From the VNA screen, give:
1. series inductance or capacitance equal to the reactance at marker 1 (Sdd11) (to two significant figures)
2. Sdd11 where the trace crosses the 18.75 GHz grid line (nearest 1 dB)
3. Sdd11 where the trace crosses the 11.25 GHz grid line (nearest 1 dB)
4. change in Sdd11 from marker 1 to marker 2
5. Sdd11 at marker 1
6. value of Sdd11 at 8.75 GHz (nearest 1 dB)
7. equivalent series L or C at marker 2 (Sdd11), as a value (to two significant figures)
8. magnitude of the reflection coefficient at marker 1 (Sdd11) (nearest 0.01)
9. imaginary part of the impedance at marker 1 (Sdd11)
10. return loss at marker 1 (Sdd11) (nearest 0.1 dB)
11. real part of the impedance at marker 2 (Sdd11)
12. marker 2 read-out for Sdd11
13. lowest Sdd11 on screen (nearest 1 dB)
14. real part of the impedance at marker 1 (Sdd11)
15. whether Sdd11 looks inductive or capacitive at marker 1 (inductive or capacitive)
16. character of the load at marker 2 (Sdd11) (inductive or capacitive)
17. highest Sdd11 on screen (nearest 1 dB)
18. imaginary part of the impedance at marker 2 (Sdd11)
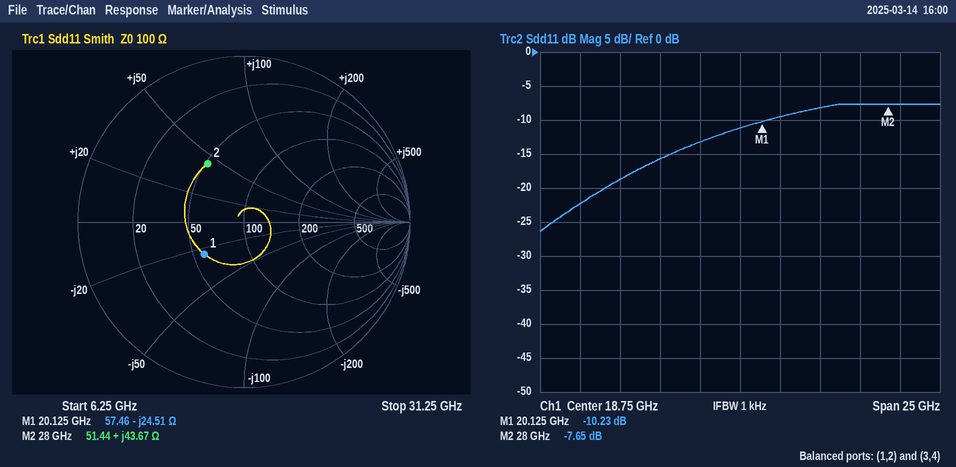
320 fF
-11 dB
-19 dB
2.58 dB
-10.23 dB
-22 dB
250 pH
0.31
-24.51 Ω
10.2 dB
51.44 Ω
-7.65 dB
-26 dB
57.46 Ω
capacitive
inductive
-8 dB
+43.67 Ω
